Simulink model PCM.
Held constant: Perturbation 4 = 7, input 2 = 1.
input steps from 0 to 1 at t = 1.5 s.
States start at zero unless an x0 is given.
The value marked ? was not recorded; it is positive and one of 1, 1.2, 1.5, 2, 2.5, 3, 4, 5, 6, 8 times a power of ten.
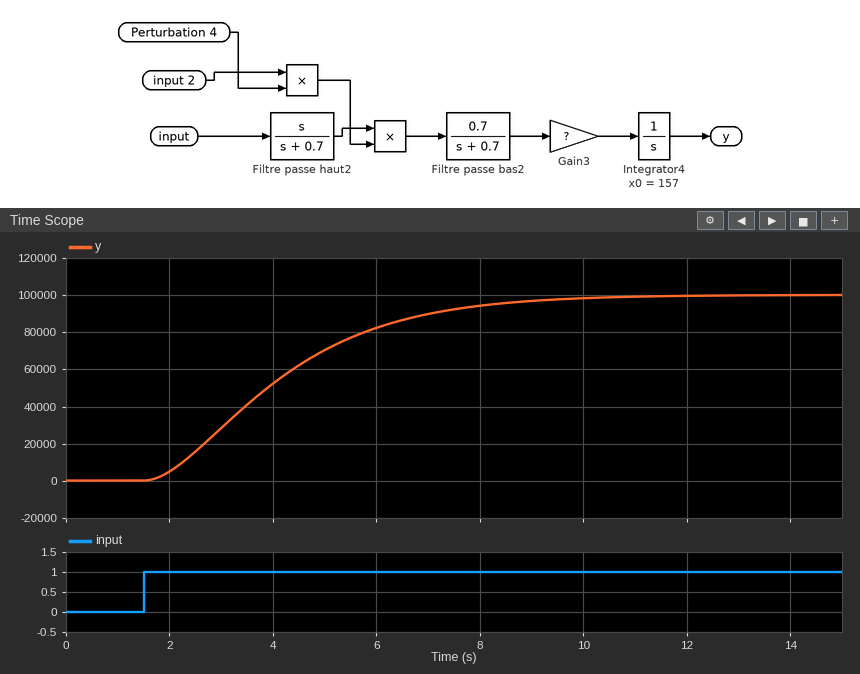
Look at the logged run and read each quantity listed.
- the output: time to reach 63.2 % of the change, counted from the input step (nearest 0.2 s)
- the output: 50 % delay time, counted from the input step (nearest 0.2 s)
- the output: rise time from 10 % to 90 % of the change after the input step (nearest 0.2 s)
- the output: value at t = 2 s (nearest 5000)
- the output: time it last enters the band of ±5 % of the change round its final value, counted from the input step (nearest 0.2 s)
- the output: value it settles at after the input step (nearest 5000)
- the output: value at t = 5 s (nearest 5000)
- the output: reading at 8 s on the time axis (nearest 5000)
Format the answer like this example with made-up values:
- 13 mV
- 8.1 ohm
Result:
- 3.0 s
- 2.4 s
- 4.8 s
- 5000
- 6.8 s
- 100000
- 70000
- 95000
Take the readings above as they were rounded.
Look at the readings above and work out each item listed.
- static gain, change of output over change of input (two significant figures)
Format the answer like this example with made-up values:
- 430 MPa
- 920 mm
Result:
- 100000
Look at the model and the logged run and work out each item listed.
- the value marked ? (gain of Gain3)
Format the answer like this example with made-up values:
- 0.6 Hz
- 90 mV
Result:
- 10000
